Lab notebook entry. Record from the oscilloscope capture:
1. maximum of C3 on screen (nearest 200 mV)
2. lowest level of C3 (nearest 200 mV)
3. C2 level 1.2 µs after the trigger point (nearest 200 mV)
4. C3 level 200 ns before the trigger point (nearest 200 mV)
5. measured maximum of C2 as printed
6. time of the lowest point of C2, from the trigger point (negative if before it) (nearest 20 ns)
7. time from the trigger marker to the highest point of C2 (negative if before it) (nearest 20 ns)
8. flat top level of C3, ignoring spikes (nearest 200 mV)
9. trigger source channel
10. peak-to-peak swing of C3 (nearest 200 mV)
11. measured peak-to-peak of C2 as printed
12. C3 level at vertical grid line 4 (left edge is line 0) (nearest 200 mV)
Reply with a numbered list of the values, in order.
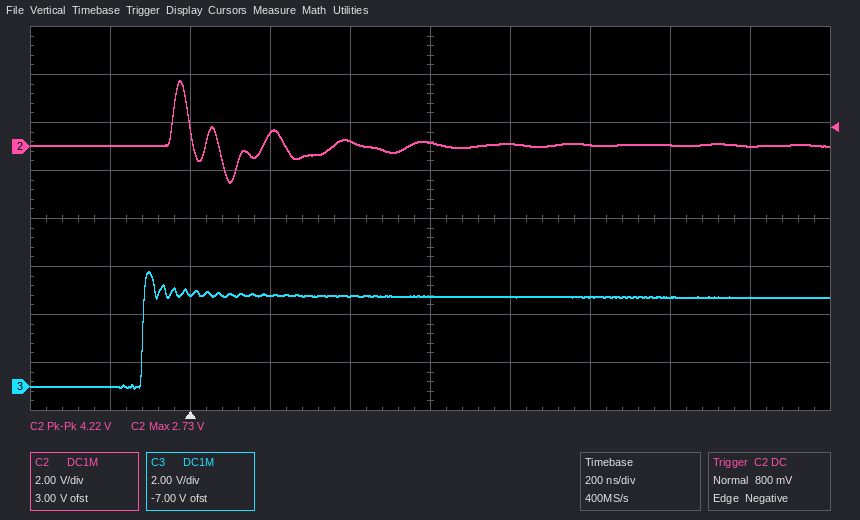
1. 4.8 V
2. 0.0 V
3. 0.0 V
4. 0.0 V
5. 2.73 V
6. +100 ns
7. -20 ns
8. 3.8 V
9. C2
10. 4.8 V
11. 4.22 V
12. 3.8 V
